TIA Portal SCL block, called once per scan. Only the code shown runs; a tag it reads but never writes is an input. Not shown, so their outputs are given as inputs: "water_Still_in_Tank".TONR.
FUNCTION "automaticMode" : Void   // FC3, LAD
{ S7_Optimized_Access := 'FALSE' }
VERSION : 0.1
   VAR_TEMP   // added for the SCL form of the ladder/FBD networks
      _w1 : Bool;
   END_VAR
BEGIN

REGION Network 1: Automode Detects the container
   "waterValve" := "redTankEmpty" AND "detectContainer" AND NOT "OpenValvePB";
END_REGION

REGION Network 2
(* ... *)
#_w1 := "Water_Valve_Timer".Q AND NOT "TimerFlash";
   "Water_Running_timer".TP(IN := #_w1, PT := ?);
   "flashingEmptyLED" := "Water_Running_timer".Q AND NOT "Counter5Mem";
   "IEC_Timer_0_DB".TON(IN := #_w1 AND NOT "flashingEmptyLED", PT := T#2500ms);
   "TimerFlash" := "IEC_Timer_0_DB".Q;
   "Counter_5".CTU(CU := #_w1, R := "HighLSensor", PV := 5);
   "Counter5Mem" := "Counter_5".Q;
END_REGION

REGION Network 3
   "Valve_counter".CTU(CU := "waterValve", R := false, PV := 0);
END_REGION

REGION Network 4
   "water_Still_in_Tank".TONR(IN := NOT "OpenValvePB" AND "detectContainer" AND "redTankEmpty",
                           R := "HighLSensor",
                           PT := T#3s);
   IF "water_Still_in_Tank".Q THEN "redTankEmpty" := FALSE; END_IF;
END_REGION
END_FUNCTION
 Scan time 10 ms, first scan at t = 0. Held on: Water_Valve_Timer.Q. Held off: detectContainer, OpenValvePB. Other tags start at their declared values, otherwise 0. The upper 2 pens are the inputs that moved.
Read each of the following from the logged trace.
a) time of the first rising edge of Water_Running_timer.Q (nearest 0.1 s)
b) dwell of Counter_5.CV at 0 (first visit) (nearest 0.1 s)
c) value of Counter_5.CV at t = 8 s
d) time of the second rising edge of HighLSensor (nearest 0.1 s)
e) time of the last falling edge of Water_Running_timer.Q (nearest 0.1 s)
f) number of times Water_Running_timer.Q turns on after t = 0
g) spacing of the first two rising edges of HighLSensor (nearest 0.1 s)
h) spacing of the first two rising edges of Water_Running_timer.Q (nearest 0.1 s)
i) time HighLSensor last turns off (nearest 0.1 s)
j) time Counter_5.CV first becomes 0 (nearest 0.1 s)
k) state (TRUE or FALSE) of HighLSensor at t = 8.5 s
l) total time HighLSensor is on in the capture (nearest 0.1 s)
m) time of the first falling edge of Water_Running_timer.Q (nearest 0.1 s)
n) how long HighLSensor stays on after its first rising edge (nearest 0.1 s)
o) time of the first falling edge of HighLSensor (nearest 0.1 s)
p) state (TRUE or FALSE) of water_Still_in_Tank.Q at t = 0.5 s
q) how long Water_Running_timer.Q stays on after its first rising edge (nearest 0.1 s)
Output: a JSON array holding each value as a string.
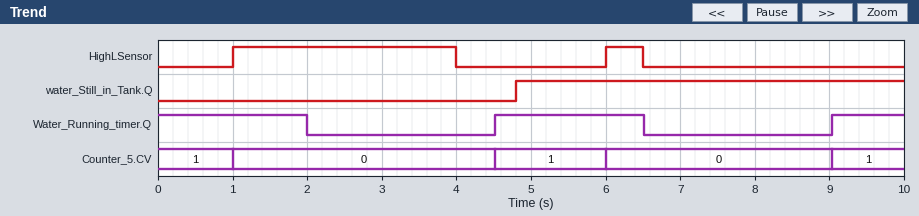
["4.5 s", "3.5 s", "0", "6.0 s", "6.5 s", "2", "5.0 s", "4.5 s", "6.5 s", "1.0 s", "FALSE", "3.5 s", "2.0 s", "3.0 s", "4.0 s", "FALSE", "2.0 s"]
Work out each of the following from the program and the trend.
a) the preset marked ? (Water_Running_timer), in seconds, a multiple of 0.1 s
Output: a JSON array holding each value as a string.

["2.0 s"]
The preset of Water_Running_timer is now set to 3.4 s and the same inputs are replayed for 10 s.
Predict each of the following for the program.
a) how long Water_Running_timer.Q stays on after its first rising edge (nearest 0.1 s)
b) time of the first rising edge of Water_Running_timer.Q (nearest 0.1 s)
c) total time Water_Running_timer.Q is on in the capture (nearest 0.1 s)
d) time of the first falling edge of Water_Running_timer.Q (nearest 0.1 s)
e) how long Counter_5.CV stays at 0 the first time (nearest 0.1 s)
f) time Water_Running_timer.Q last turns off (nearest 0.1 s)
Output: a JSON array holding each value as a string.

["3.4 s", "5.9 s", "6.8 s", "3.4 s", "4.9 s", "9.3 s"]
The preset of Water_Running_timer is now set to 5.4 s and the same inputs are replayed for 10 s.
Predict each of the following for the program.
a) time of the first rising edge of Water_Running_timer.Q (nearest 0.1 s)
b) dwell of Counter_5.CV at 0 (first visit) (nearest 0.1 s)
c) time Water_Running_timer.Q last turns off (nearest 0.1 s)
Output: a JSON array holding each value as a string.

["7.9 s", "6.9 s", "5.4 s"]
